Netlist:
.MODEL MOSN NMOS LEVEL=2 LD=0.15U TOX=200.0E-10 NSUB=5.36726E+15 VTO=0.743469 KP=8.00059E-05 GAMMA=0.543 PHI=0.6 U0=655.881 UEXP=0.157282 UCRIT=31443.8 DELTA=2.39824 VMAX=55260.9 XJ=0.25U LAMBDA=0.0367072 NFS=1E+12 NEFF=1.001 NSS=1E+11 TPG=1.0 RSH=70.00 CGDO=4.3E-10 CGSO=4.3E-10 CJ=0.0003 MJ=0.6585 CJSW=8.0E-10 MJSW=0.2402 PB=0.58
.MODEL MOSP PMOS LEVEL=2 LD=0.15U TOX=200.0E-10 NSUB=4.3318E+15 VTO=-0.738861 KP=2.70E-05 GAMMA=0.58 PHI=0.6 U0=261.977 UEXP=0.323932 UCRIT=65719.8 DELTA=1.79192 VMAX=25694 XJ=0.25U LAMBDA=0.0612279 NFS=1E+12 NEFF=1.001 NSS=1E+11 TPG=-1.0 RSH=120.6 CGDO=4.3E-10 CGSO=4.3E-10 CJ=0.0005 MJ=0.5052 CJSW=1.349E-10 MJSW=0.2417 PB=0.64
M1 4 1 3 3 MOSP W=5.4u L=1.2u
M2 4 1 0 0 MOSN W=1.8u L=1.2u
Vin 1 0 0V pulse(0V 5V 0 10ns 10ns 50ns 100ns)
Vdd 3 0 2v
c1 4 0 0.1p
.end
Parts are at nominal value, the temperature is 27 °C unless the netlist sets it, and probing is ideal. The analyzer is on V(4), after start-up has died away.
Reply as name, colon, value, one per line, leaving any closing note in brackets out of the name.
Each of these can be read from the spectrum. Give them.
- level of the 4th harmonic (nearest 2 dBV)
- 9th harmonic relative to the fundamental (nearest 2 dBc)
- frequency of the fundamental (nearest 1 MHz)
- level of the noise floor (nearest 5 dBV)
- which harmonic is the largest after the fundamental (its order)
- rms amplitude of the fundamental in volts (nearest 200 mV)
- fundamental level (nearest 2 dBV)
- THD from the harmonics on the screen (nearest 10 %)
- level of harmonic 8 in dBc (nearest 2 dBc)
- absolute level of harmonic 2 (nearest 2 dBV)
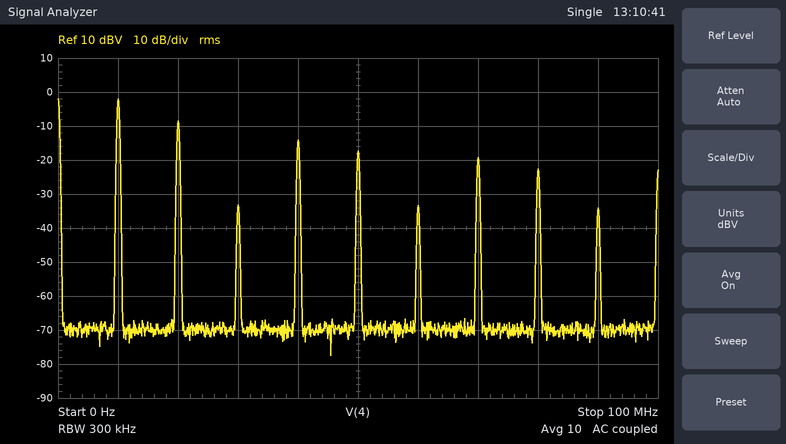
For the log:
level of the 4th harmonic: -14 dBV
9th harmonic relative to the fundamental: -32 dBc
frequency of the fundamental: 10 MHz
level of the noise floor: -70 dBV
which harmonic is the largest after the fundamental: 2
rms amplitude of the fundamental in volts: 800 mV
fundamental level: -2 dBV
THD from the harmonics on the screen: 60 %
level of harmonic 8 in dBc: -20 dBc
absolute level of harmonic 2: -8 dBV
